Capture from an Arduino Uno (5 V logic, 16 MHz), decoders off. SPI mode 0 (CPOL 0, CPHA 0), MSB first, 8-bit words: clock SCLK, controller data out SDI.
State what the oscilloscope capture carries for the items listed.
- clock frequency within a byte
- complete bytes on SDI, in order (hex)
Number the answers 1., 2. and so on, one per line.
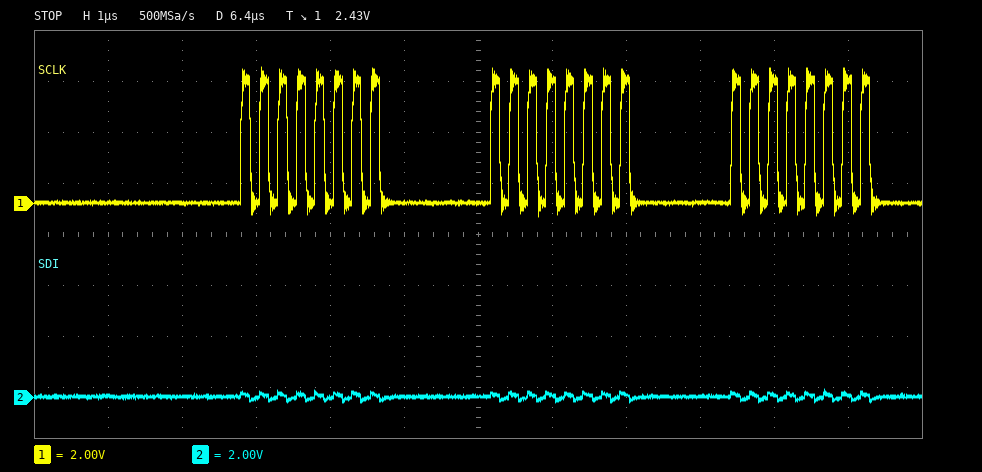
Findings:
1. 4 MHz
2. 00 00 00
